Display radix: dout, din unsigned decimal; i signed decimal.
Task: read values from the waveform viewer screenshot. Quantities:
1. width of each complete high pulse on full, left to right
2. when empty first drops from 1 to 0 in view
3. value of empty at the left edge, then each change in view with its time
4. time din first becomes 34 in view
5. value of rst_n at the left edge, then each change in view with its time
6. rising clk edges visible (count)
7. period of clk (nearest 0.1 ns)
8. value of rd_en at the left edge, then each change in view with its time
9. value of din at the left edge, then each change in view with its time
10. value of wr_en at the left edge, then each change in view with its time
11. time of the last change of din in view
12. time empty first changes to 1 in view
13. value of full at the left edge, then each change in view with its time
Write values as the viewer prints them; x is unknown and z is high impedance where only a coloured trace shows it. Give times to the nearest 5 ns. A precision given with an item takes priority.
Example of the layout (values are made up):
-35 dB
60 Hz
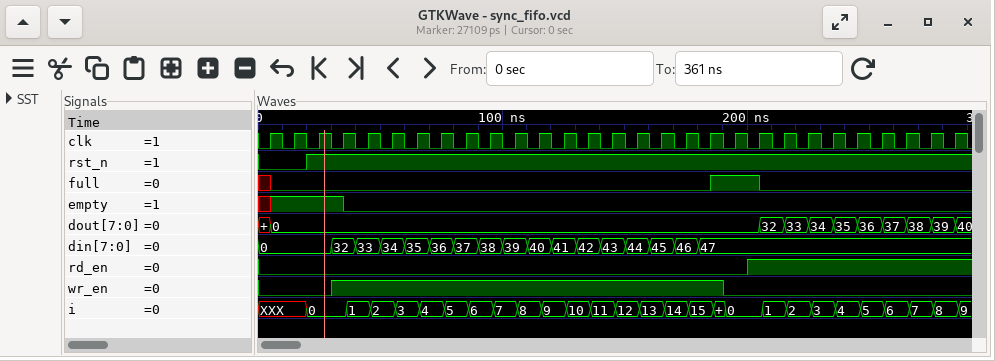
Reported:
20 ns
35 ns
x, 1 at 5 ns, 0 at 35 ns
50 ns
0, 1 at 20 ns
29
10 ns
0, 1 at 200 ns
0, 32 at 30 ns, 33 at 40 ns, 34 at 50 ns, 35 at 60 ns, 36 at 70 ns, 37 at 80 ns, 38 at 90 ns, 39 at 100 ns, 40 at 110 ns, 41 at 120 ns, 42 at 130 ns, 43 at 140 ns, 44 at 150 ns, 45 at 160 ns, 46 at 170 ns, 47 at 180 ns
0, 1 at 30 ns, 0 at 190 ns
180 ns
5 ns
x, 0 at 5 ns, 1 at 185 ns, 0 at 205 ns
